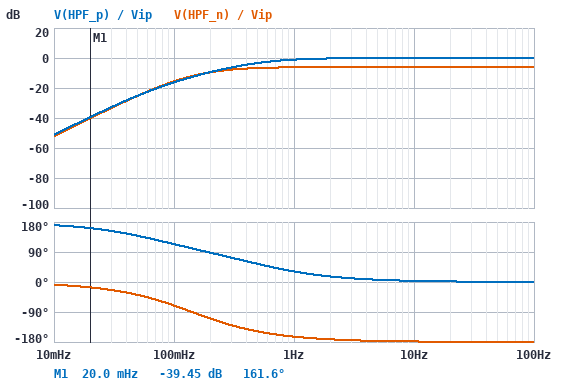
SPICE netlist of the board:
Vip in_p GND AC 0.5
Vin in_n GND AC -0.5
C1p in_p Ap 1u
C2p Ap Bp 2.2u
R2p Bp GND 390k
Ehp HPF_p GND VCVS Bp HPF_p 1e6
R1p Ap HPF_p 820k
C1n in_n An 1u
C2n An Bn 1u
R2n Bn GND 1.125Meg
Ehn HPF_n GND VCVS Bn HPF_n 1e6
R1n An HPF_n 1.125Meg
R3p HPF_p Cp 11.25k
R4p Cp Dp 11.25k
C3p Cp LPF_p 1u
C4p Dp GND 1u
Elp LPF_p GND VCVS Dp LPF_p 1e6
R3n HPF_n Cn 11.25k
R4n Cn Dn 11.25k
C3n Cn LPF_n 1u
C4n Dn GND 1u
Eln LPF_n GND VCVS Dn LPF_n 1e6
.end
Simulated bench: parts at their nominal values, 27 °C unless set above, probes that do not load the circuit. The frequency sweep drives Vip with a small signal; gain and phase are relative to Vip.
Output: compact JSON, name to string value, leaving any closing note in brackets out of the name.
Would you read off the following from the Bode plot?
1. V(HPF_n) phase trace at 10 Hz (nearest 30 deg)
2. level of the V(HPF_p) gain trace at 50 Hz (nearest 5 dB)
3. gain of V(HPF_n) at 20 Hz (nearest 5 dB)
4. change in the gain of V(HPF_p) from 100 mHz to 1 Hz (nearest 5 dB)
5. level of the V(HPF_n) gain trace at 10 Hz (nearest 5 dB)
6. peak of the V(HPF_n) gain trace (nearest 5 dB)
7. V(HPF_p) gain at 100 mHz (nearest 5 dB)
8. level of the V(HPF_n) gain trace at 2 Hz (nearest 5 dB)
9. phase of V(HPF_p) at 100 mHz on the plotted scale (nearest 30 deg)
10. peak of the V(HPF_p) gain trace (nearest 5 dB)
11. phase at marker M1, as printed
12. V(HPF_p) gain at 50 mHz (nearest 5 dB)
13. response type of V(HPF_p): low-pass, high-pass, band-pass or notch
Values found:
{"V(HPF_n) phase trace at 10 Hz": "-180 deg", "level of the V(HPF_p) gain trace at 50 Hz": "0 dB", "gain of V(HPF_n) at 20 Hz": "-5 dB", "change in the gain of V(HPF_p) from 100 mHz to 1 Hz": "15 dB", "level of the V(HPF_n) gain trace at 10 Hz": "-5 dB", "peak of the V(HPF_n) gain trace": "-5 dB", "V(HPF_p) gain at 100 mHz": "-15 dB", "level of the V(HPF_n) gain trace at 2 Hz": "-5 dB", "phase of V(HPF_p) at 100 mHz on the plotted scale": "120 deg", "peak of the V(HPF_p) gain trace": "0 dB", "phase at marker M1, as printed": "161.6 deg", "V(HPF_p) gain at 50 mHz": "-25 dB", "response type of V(HPF_p): low-pass, high-pass, band-pass or notch": "high-pass"}
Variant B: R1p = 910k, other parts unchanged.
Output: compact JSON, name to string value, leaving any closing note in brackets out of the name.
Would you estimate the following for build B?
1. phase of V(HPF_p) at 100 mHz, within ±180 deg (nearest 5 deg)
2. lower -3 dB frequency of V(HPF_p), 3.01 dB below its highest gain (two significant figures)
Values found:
{"phase of V(HPF_p) at 100 mHz, within ±180 deg": "110 deg", "lower -3 dB frequency of V(HPF_p), 3.01 dB below its highest gain": "540 mHz"}
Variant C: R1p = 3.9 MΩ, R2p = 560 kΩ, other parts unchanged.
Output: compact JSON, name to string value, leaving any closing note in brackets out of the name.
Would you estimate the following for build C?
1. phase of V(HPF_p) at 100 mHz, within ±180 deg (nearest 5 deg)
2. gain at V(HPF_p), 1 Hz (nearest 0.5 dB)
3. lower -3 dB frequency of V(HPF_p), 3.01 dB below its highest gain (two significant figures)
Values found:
{"phase of V(HPF_p) at 100 mHz, within ±180 deg": "85 deg", "gain at V(HPF_p), 1 Hz": "-0.5 dB", "lower -3 dB frequency of V(HPF_p), 3.01 dB below its highest gain": "400 mHz"}
